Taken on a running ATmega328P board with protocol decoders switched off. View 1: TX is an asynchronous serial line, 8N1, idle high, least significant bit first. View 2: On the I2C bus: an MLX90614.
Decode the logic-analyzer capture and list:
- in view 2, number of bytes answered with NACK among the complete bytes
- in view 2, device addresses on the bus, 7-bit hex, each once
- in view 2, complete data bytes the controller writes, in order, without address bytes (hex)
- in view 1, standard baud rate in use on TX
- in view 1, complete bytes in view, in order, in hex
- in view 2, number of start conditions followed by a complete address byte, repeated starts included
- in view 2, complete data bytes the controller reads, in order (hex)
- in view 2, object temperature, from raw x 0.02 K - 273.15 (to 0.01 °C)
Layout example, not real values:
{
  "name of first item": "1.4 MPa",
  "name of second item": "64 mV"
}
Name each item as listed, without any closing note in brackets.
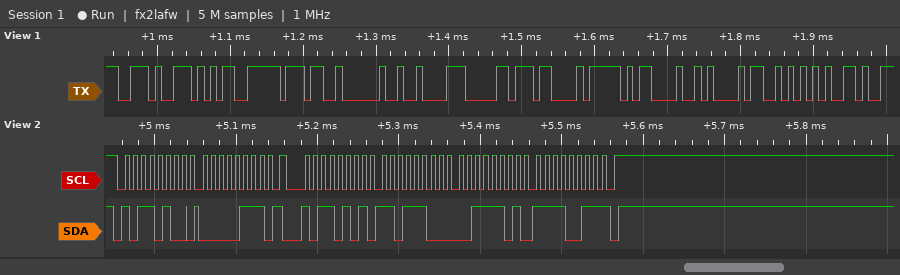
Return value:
{
  "in view 2, number of bytes answered with NACK among the complete bytes": "1",
  "in view 2, device addresses on the bus, 7-bit hex, each once": "0x5A",
  "in view 2, complete data bytes the controller writes, in order, without address bytes": "07",
  "in view 1, standard baud rate in use on TX": "115200 baud",
  "in view 1, complete bytes in view, in order, in hex": "0x2E 0x35 0x37 0x20 0xC2 0xB0 0x43 0x0D 0x0A 0x53 0x65",
  "in view 2, number of start conditions followed by a complete address byte, repeated starts included": "2",
  "in view 2, complete data bytes the controller reads, in order": "DC 3D F3",
  "in view 2, object temperature, from raw x 0.02 K - 273.15": "43.57 °C"
}
